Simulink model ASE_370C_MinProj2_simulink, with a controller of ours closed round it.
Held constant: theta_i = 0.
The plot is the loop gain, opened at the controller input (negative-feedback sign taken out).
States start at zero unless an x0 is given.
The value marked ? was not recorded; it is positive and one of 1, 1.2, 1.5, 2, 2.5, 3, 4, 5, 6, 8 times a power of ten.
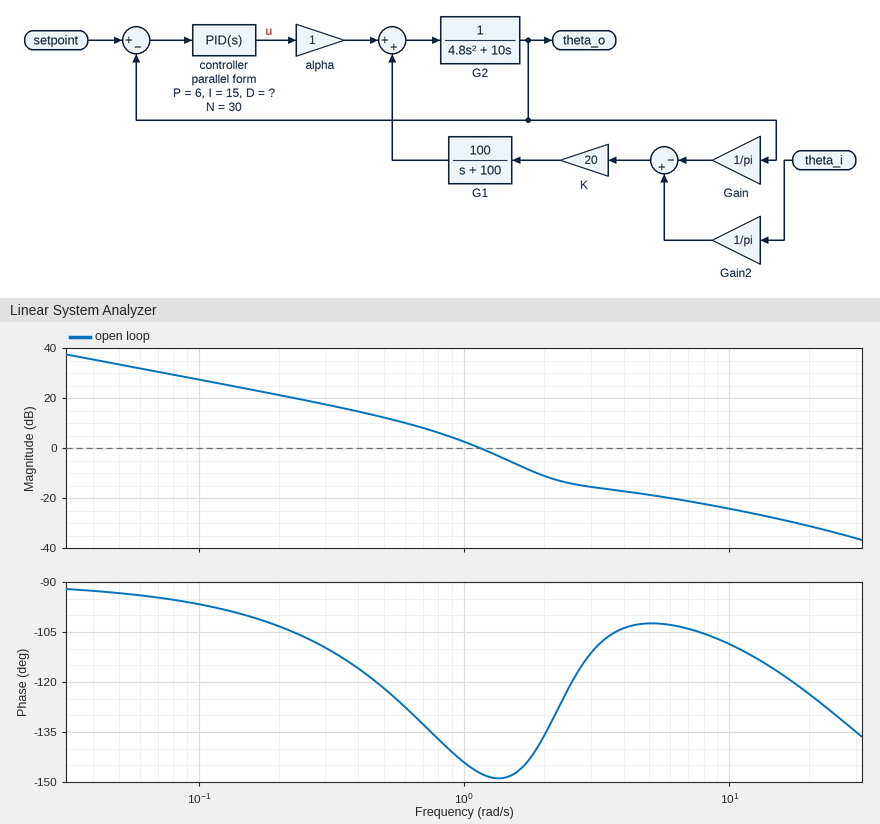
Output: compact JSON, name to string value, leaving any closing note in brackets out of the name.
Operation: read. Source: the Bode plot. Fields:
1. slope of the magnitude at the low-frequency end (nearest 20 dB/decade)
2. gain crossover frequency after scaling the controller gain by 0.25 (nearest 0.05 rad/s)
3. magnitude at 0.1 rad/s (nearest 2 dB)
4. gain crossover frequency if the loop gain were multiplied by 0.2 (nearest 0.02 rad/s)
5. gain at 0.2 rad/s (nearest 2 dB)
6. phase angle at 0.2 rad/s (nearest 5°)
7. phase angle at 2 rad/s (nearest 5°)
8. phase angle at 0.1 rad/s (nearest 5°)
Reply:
{"slope of the magnitude at the low-frequency end": "-20 dB/decade", "gain crossover frequency after scaling the controller gain by 0.25": "0.50 rad/s", "magnitude at 0.1 rad/s": "28 dB", "gain crossover frequency if the loop gain were multiplied by 0.2": "0.42 rad/s", "gain at 0.2 rad/s": "22 dB", "phase angle at 0.2 rad/s": "-105°", "phase angle at 2 rad/s": "-135°", "phase angle at 0.1 rad/s": "-95°"}
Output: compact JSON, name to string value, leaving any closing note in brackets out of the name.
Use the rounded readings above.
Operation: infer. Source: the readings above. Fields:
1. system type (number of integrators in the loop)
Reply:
{"system type": "1"}
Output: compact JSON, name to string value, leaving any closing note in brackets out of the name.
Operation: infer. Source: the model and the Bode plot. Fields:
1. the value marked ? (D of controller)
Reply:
{"the value marked ?": "3"}
